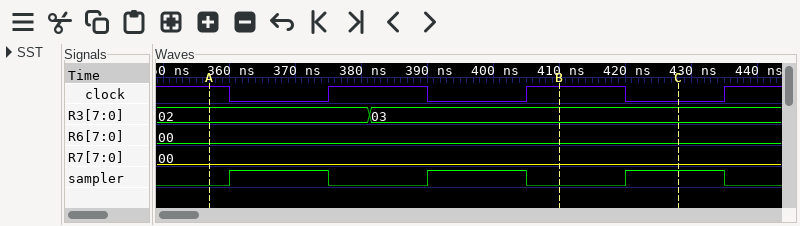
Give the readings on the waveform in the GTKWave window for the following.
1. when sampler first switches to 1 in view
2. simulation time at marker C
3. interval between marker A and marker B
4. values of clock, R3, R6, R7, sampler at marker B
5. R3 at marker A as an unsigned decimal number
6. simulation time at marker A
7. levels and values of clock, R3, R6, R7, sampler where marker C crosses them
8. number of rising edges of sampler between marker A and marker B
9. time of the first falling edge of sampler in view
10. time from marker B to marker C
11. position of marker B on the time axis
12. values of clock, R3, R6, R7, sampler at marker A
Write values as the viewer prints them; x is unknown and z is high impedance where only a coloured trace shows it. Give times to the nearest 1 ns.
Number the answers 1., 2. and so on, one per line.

1. 360 ns
2. 428 ns
3. 53 ns
4. clock=1, R3=03, R6=00, R7=00, sampler=0
5. 2
6. 357 ns
7. clock=0, R3=03, R6=00, R7=00, sampler=1
8. 2
9. 375 ns
10. 18 ns
11. 410 ns
12. clock=1, R3=02, R6=00, R7=00, sampler=0
